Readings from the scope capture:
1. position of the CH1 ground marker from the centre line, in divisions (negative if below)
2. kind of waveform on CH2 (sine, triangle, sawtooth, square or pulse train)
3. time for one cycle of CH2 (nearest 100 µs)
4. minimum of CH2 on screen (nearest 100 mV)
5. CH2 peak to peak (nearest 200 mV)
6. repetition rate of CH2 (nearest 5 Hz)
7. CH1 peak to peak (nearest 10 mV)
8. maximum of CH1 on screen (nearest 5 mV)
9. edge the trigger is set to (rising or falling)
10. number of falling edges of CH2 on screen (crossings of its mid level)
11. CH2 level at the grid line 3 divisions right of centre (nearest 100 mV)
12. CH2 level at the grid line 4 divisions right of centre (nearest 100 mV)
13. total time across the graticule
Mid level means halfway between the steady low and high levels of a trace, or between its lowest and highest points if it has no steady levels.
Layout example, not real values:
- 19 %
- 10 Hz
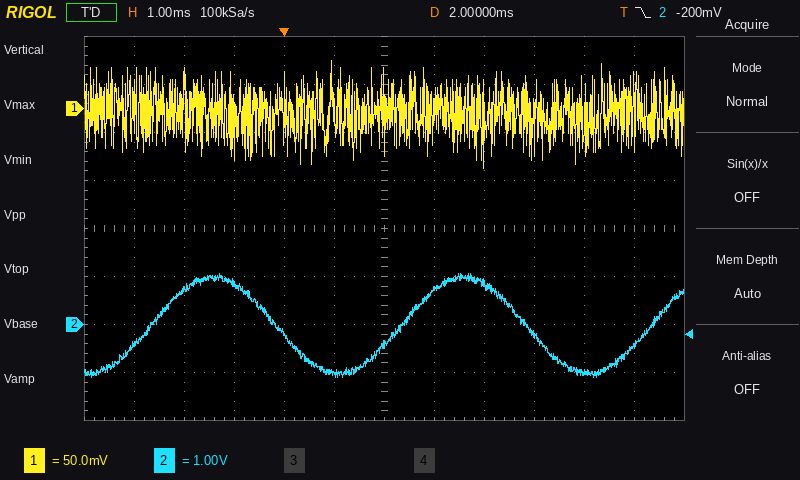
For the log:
- +2.5 div
- sine
- 5.0 ms
- -1.1 V
- 2.2 V
- 200 Hz
- 110 mV
- 50 mV
- falling
- 2
- -200 mV
- -1.0 V
- 12 ms
